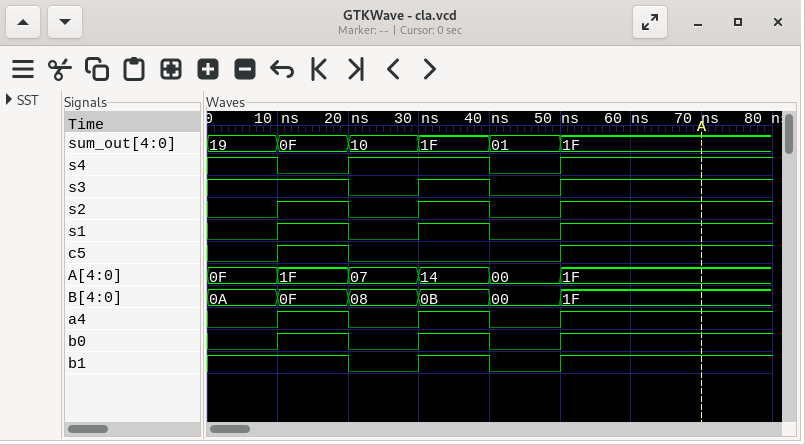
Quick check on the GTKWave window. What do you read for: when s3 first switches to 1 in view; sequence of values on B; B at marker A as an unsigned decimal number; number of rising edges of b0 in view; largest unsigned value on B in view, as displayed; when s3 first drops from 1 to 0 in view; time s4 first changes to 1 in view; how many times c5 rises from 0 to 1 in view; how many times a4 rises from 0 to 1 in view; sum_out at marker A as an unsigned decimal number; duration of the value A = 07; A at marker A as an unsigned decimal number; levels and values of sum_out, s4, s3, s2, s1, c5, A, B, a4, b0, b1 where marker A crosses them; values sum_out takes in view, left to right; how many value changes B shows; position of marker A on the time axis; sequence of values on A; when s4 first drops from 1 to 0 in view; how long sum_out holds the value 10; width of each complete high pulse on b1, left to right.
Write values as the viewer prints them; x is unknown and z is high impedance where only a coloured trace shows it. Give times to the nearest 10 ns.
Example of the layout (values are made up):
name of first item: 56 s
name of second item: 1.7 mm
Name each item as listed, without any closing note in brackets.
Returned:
when s3 first switches to 1 in view: 30 ns
sequence of values on B: 0A, 0F, 08, 0B, 00, 1F
B at marker A as an unsigned decimal number: 31
number of rising edges of b0 in view: 3
largest unsigned value on B in view, as displayed: 1F
when s3 first drops from 1 to 0 in view: 20 ns
time s4 first changes to 1 in view: 20 ns
how many times c5 rises from 0 to 1 in view: 2
how many times a4 rises from 0 to 1 in view: 3
sum_out at marker A as an unsigned decimal number: 31
duration of the value A = 07: 10 ns
A at marker A as an unsigned decimal number: 31
levels and values of sum_out, s4, s3, s2, s1, c5, A, B, a4, b0, b1 where marker A crosses them: sum_out=1F, s4=1, s3=1, s2=1, s1=1, c5=1, A=1F, B=1F, a4=1, b0=1, b1=1
values sum_out takes in view, left to right: 19, 0F, 10, 1F, 01, 1F
how many value changes B shows: 5
position of marker A on the time axis: 70 ns
sequence of values on A: 0F, 1F, 07, 14, 00, 1F
when s4 first drops from 1 to 0 in view: 10 ns
how long sum_out holds the value 10: 10 ns
width of each complete high pulse on b1, left to right: 10 ns
